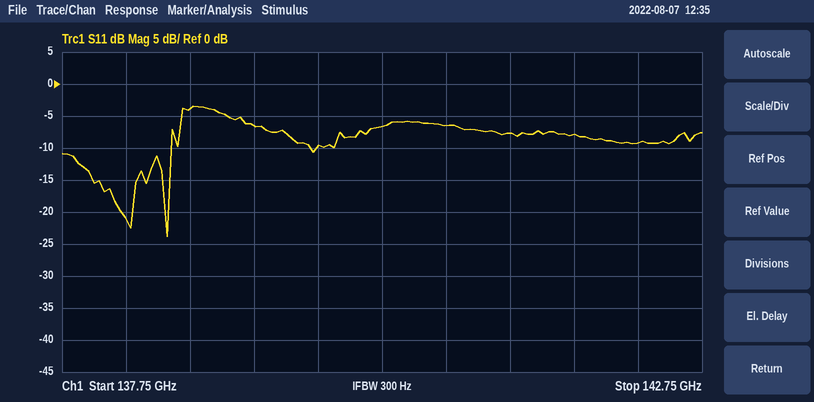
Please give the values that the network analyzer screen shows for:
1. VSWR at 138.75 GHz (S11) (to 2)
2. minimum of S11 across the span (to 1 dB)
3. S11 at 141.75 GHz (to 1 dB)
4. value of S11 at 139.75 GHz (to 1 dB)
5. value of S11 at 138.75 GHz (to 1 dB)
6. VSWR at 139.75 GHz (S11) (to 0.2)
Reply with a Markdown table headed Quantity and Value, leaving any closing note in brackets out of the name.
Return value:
| Quantity | Value |
|---|---|
| VSWR at 138.75 GHz (S11) | 4 |
| minimum of S11 across the span | -24 dB |
| S11 at 141.75 GHz | -8 dB |
| value of S11 at 139.75 GHz | -10 dB |
| value of S11 at 138.75 GHz | -4 dB |
| VSWR at 139.75 GHz (S11) | 2.0 |
